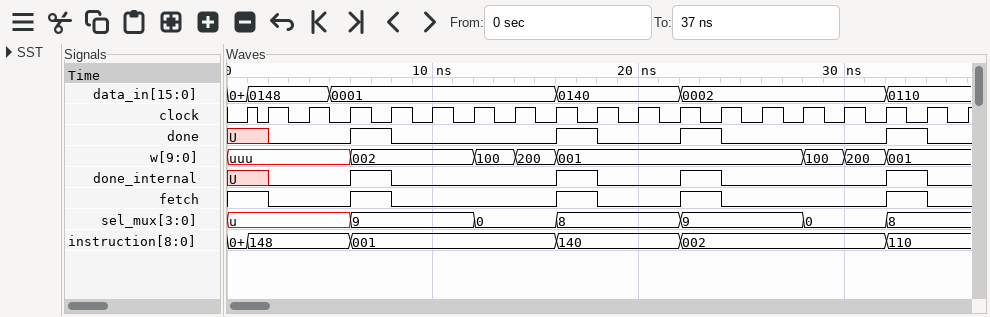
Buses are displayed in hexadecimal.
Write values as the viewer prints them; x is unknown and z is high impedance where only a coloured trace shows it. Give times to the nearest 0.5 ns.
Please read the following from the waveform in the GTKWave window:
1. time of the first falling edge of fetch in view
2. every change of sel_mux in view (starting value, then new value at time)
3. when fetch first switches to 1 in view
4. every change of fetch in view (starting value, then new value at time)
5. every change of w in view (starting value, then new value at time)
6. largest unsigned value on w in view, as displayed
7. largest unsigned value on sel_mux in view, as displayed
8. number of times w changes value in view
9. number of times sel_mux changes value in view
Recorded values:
2 ns
u, 9 at 6 ns, 0 at 12 ns, 8 at 16 ns, 9 at 22 ns, 0 at 28 ns, 8 at 32 ns
6 ns
1, 0 at 2 ns, 1 at 6 ns, 0 at 8 ns, 1 at 16 ns, 0 at 18 ns, 1 at 22 ns, 0 at 24 ns, 1 at 32 ns, 0 at 34 ns
uuu, 002 at 6 ns, 100 at 12 ns, 200 at 14 ns, 001 at 16 ns, 100 at 28 ns, 200 at 30 ns, 001 at 32 ns
200
9
7
6
